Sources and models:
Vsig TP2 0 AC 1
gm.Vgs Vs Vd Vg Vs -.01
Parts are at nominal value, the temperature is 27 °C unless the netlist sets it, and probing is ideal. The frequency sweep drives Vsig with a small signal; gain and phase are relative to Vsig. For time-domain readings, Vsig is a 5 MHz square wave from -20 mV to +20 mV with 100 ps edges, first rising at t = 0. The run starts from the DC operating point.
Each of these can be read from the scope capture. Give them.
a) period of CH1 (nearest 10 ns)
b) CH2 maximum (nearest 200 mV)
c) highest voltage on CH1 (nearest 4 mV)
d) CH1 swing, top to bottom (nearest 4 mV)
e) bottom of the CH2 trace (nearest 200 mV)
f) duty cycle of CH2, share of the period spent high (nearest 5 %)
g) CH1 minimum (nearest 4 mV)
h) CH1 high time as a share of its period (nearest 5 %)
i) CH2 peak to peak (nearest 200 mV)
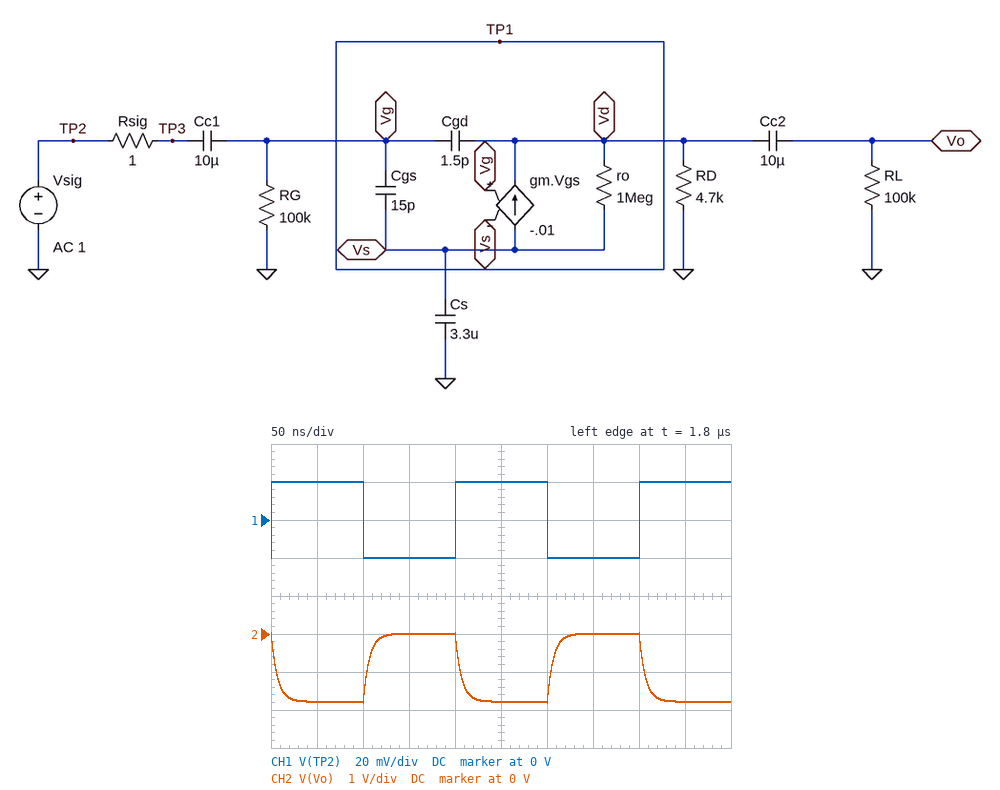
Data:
200 ns
0 V
20 mV
40 mV
-1.8 V
50 %
-20 mV
50 %
1.8 V
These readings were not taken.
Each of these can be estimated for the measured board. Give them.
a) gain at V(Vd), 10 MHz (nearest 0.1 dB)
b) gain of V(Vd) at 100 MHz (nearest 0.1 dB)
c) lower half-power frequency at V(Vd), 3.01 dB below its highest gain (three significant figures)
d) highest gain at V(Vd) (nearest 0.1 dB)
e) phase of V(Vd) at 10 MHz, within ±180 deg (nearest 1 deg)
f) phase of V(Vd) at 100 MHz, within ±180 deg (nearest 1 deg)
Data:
32.3 dB
20.2 dB
480 Hz
33.0 dB
156 deg
97 deg
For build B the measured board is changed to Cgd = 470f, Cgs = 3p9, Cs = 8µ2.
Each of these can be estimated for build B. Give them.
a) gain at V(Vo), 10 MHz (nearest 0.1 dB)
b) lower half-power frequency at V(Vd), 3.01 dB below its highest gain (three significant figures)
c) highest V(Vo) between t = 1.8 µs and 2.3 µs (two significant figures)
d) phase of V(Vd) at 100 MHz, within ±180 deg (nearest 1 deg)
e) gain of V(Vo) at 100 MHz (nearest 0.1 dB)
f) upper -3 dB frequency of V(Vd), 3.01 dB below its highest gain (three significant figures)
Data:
32.9 dB
193 Hz
11 mV
125 deg
28.6 dB
75.0 MHz
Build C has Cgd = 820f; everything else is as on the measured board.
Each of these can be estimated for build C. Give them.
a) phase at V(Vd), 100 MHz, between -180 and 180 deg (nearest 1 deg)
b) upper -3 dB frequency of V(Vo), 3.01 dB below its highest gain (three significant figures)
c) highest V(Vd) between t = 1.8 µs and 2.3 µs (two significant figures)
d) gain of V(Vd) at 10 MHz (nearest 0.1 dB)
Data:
110 deg
43.0 MHz
21 mV
32.8 dB
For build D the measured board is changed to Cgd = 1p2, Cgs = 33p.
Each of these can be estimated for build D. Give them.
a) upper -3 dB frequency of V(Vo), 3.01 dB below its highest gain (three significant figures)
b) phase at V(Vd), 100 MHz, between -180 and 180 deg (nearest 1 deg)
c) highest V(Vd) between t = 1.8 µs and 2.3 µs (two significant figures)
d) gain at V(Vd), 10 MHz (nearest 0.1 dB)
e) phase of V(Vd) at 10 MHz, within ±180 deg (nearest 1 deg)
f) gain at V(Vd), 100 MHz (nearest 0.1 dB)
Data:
29.4 MHz
101 deg
25 mV
32.5 dB
161 deg
22.0 dB
